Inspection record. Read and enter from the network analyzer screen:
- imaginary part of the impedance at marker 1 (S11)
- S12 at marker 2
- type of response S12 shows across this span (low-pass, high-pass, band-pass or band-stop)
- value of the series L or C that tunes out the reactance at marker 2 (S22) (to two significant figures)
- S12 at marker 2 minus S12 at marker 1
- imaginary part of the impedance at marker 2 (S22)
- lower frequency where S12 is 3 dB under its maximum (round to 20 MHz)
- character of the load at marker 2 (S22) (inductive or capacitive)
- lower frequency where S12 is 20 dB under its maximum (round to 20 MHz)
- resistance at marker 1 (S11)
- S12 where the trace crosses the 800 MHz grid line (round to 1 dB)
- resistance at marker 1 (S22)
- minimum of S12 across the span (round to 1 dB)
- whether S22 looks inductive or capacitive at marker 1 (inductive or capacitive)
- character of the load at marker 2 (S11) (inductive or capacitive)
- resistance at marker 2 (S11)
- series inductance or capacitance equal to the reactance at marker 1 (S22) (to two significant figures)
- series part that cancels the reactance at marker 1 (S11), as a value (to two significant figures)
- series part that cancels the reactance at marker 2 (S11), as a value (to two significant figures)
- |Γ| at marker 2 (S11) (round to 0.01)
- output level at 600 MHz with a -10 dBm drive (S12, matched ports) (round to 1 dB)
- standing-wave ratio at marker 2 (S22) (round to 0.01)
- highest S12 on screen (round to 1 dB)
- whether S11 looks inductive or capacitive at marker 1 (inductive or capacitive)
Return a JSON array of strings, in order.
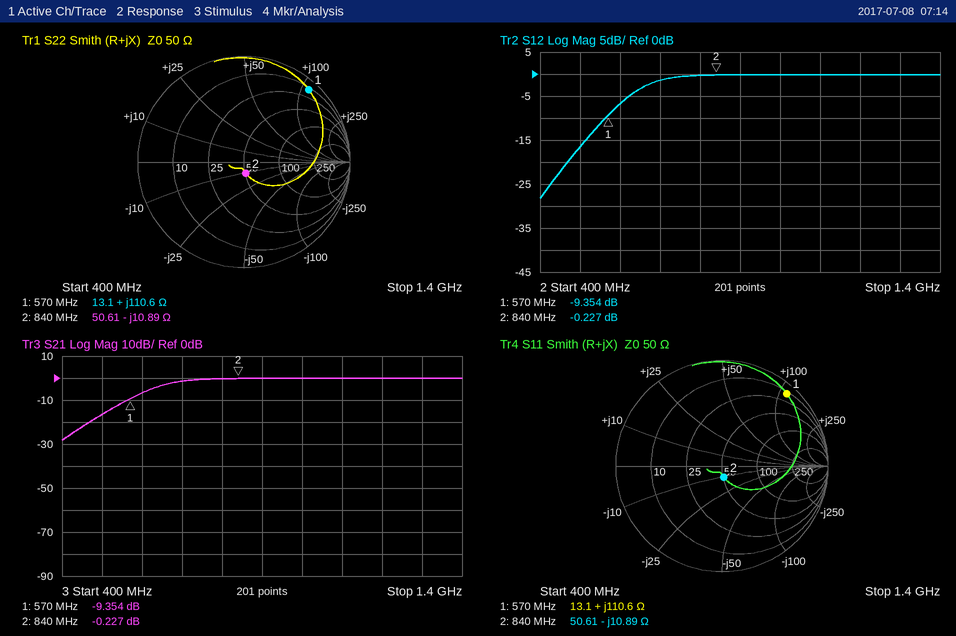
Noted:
["+110.6 Ω", "-0.227 dB", "high-pass", "2.1 nH", "9.127 dB", "-10.89 Ω", "660 MHz", "capacitive", "460 MHz", "13.1 Ω", "0 dB", "13.1 Ω", "-28 dB", "inductive", "capacitive", "50.61 Ω", "31 nH", "2.5 pF", "2.1 nH", "0.11", "-17 dBm", "1.24", "0 dB", "inductive"]
